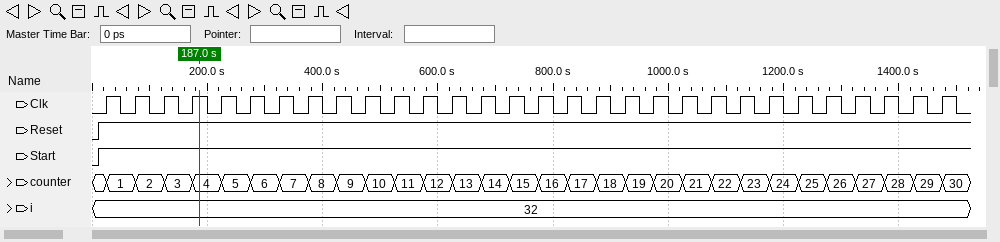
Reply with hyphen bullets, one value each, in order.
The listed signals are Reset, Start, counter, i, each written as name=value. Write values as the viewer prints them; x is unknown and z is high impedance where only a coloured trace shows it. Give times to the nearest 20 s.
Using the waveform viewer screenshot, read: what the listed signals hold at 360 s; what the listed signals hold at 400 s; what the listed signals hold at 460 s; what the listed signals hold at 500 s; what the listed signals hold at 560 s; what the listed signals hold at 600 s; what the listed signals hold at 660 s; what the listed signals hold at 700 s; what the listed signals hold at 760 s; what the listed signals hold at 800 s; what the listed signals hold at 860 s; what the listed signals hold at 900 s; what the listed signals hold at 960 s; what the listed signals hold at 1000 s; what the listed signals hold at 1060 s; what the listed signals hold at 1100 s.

- Reset=1, Start=1, counter=7, i=32
- Reset=1, Start=1, counter=8, i=32
- Reset=1, Start=1, counter=9, i=32
- Reset=1, Start=1, counter=10, i=32
- Reset=1, Start=1, counter=11, i=32
- Reset=1, Start=1, counter=12, i=32
- Reset=1, Start=1, counter=13, i=32
- Reset=1, Start=1, counter=14, i=32
- Reset=1, Start=1, counter=15, i=32
- Reset=1, Start=1, counter=16, i=32
- Reset=1, Start=1, counter=17, i=32
- Reset=1, Start=1, counter=18, i=32
- Reset=1, Start=1, counter=19, i=32
- Reset=1, Start=1, counter=20, i=32
- Reset=1, Start=1, counter=21, i=32
- Reset=1, Start=1, counter=22, i=32
